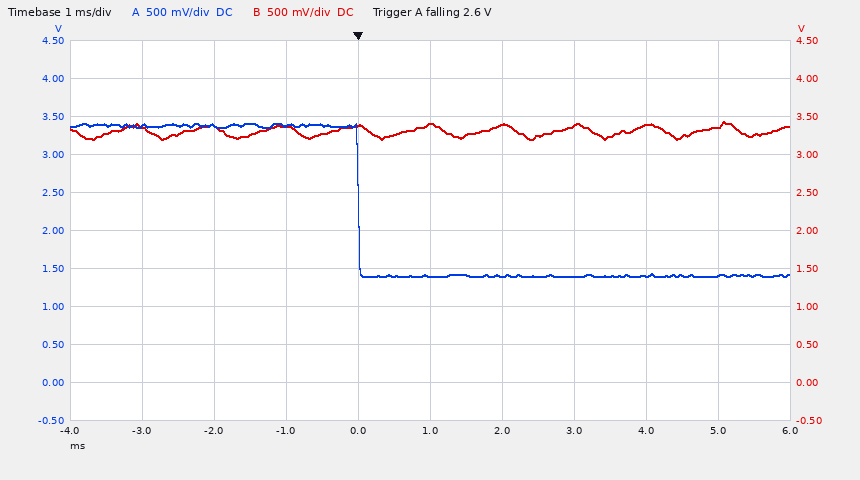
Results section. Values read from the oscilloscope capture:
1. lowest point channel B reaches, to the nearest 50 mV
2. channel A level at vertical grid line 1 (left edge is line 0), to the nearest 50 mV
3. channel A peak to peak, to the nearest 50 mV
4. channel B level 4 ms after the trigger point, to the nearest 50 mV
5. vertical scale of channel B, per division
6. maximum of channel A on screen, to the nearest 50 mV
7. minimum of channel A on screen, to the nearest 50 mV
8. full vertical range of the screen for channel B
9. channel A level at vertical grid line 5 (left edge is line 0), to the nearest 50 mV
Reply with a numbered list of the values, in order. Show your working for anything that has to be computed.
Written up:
1. 3.20 V
2. 3.40 V
3. 3.40 V − (1.40 V) = 2.00 V
4. 3.40 V
5. 500 mV
6. 3.40 V
7. 1.40 V
8. 5 V
9. 1.40 V
